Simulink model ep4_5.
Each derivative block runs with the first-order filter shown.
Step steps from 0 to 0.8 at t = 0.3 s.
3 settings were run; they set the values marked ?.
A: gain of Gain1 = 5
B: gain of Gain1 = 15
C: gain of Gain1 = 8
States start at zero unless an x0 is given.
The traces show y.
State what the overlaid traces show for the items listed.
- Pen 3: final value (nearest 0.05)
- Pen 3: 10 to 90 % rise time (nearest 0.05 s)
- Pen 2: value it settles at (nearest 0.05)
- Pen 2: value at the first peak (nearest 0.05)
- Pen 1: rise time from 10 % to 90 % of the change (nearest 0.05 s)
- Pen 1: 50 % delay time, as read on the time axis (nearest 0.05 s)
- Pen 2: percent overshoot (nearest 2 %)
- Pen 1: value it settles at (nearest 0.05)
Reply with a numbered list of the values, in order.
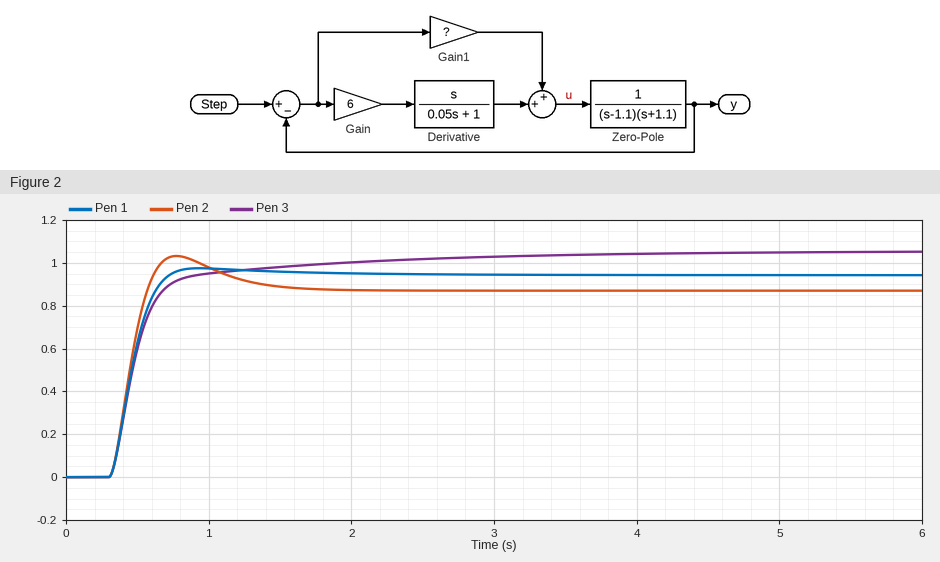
1. 1.05
2. 0.65 s
3. 0.85
4. 1.05
5. 0.25 s
6. 0.45 s
7. 18 %
8. 0.95
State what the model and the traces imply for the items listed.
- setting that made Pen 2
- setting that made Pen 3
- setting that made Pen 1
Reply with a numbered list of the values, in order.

1. B
2. A
3. C
